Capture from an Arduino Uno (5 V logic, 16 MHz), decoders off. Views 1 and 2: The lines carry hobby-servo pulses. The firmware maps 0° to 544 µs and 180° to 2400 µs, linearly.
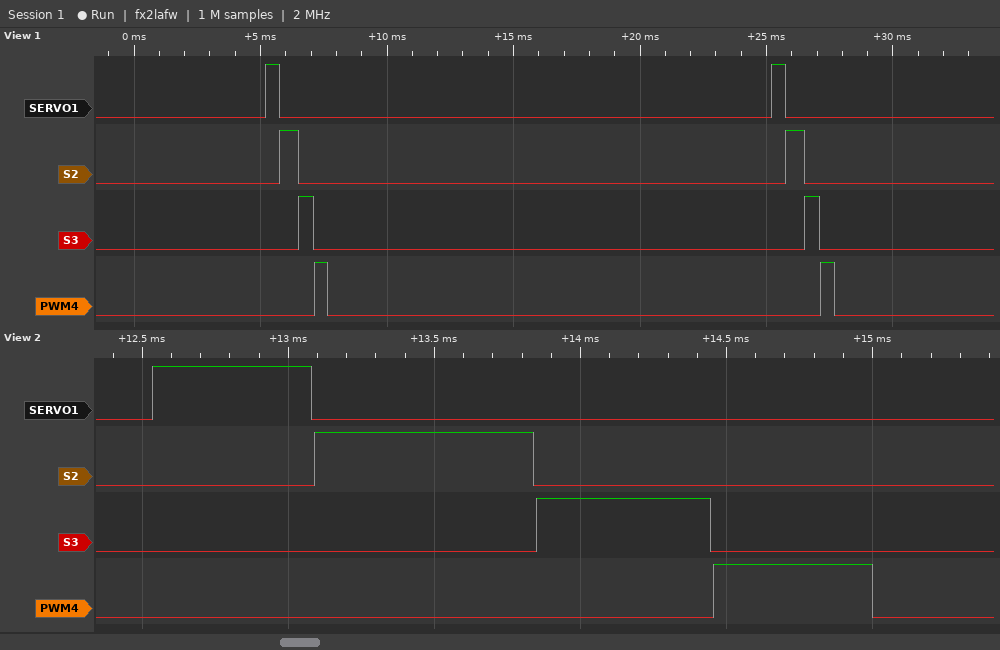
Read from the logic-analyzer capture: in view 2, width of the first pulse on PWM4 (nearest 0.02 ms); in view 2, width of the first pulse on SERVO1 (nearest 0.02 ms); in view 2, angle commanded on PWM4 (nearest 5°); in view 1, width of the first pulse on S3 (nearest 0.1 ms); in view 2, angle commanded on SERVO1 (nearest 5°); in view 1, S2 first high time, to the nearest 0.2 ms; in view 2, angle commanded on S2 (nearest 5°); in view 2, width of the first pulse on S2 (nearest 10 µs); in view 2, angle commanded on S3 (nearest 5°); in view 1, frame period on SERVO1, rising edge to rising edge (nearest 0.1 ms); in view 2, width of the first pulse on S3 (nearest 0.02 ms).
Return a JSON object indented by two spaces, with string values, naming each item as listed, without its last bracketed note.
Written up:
{
  "in view 2, width of the first pulse on PWM4": "0.54 ms",
  "in view 2, width of the first pulse on SERVO1": "0.54 ms",
  "in view 2, angle commanded on PWM4": "0°",
  "in view 1, width of the first pulse on S3": "0.6 ms",
  "in view 2, angle commanded on SERVO1": "0°",
  "in view 1, S2 first high time, to the nearest 0.2 ms": "0.8 ms",
  "in view 2, angle commanded on S2": "20°",
  "in view 2, width of the first pulse on S2": "750 µs",
  "in view 2, angle commanded on S3": "5°",
  "in view 1, frame period on SERVO1, rising edge to rising edge": "20.0 ms",
  "in view 2, width of the first pulse on S3": "0.60 ms"
}
